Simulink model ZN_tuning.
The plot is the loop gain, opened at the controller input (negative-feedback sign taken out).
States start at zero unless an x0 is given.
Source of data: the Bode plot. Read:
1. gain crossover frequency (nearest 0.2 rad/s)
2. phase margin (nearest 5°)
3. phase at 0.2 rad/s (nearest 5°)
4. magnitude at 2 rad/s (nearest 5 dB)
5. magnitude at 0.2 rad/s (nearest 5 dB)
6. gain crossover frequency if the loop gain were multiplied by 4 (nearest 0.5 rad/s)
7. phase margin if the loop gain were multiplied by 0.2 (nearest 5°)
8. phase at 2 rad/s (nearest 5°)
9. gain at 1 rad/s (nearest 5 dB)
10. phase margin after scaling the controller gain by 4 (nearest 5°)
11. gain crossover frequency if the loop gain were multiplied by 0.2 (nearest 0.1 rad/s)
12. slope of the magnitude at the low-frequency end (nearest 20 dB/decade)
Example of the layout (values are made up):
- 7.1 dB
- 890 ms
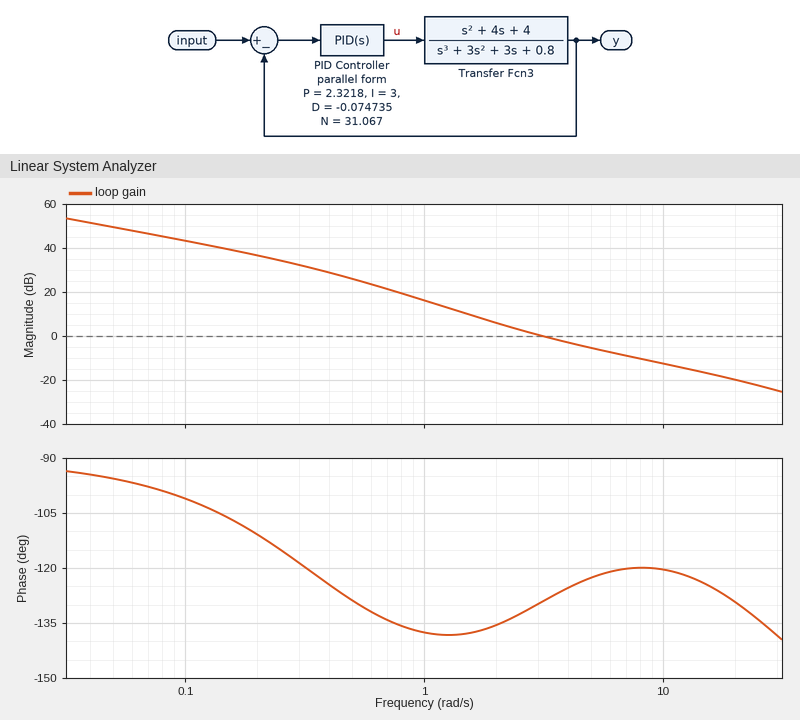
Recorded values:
- 3.2 rad/s
- 50°
- -110°
- 5 dB
- 35 dB
- 9.5 rad/s
- 40°
- -135°
- 15 dB
- 60°
- 1.2 rad/s
- -20 dB/decade
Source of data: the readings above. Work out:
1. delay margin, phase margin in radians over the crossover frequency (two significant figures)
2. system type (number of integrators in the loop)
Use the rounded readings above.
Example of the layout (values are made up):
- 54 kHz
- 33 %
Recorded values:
- 0.27 s
- 1
